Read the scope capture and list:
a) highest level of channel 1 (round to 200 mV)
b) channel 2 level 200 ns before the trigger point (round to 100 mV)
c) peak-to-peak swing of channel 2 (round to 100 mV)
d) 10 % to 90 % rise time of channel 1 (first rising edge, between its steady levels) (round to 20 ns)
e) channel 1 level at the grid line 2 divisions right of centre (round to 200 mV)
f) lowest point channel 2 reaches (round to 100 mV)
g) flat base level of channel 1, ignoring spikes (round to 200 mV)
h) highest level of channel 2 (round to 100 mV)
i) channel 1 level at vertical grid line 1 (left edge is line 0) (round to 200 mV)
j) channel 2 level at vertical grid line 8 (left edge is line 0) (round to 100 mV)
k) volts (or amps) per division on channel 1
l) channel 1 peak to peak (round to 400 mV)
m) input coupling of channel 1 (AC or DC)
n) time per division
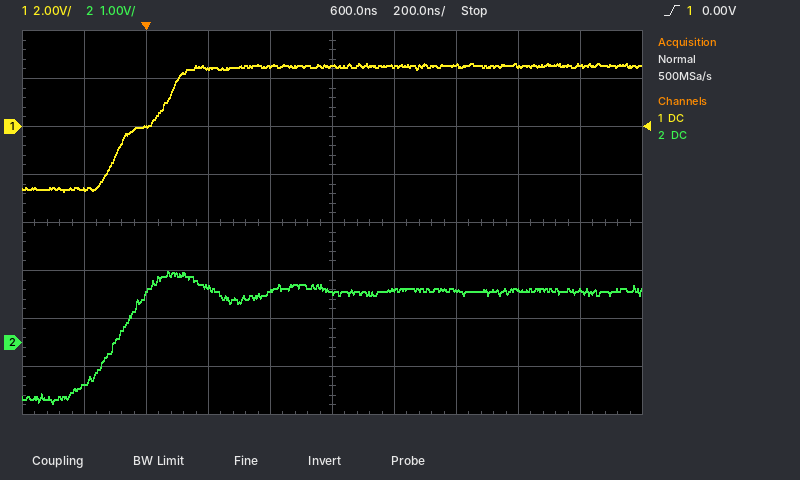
2.6 V
-900 mV
2.8 V
240 ns
2.6 V
-1.3 V
-2.6 V
1.5 V
-2.6 V
1.1 V
2 V
5.2 V
DC
200 ns
